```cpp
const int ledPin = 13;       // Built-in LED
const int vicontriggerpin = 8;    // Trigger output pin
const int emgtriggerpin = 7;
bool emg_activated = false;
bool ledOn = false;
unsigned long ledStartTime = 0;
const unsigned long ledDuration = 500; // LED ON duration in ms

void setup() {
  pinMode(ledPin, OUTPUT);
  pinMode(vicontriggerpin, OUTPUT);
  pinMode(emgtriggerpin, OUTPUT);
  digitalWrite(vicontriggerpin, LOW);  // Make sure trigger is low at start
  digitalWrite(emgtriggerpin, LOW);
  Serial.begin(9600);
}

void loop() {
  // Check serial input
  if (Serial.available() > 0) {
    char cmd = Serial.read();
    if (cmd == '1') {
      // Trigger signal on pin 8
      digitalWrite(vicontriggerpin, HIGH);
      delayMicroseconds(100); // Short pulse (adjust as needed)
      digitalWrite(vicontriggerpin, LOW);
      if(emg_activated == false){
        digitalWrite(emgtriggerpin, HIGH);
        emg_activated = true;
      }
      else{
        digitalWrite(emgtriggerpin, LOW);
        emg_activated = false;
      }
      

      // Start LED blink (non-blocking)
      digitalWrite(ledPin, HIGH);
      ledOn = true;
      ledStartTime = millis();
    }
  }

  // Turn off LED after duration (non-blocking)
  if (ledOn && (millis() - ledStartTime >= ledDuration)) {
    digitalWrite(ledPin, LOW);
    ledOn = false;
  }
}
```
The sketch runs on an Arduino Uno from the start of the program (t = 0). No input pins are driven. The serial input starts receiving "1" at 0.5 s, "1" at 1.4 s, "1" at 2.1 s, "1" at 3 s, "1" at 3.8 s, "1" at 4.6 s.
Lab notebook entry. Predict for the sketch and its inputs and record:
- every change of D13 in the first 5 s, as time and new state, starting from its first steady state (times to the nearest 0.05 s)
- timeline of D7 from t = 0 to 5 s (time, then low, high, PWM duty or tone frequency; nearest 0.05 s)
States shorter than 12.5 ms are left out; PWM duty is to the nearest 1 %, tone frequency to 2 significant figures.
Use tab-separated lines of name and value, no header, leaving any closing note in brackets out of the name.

every change of D13 in the first 5 s, as time and new state, starting from its first steady state	0 s low; 0.5 s high; 1 s low; 1.4 s high; 1.9 s low; 2.1 s high; 2.6 s low; 3 s high; 3.5 s low; 3.8 s high; 4.3 s low; 4.6 s high
timeline of D7 from t = 0 to 5 s	0 s low; 0.5 s high; 1.4 s low; 2.1 s high; 3 s low; 3.8 s high; 4.6 s low
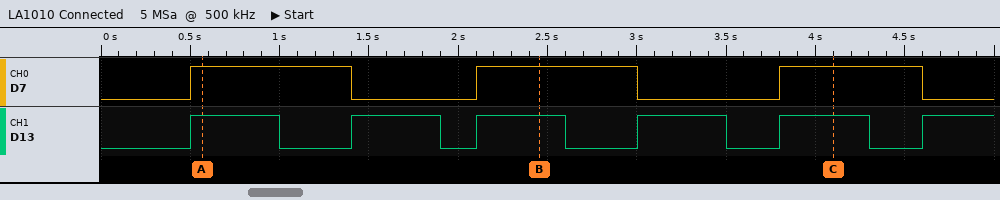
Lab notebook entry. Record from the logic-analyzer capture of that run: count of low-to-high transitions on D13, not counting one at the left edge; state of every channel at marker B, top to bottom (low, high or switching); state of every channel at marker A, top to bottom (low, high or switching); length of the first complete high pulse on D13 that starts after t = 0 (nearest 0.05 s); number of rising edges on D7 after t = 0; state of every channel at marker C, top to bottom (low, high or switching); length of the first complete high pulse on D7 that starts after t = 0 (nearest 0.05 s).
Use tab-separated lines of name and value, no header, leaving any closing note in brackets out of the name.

count of low-to-high transitions on D13, not counting one at the left edge	6
state of every channel at marker B, top to bottom	D7 high, D13 high
state of every channel at marker A, top to bottom	D7 high, D13 high
length of the first complete high pulse on D13 that starts after t = 0	0.50 s
number of rising edges on D7 after t = 0	3
state of every channel at marker C, top to bottom	D7 high, D13 high
length of the first complete high pulse on D7 that starts after t = 0	0.90 s
